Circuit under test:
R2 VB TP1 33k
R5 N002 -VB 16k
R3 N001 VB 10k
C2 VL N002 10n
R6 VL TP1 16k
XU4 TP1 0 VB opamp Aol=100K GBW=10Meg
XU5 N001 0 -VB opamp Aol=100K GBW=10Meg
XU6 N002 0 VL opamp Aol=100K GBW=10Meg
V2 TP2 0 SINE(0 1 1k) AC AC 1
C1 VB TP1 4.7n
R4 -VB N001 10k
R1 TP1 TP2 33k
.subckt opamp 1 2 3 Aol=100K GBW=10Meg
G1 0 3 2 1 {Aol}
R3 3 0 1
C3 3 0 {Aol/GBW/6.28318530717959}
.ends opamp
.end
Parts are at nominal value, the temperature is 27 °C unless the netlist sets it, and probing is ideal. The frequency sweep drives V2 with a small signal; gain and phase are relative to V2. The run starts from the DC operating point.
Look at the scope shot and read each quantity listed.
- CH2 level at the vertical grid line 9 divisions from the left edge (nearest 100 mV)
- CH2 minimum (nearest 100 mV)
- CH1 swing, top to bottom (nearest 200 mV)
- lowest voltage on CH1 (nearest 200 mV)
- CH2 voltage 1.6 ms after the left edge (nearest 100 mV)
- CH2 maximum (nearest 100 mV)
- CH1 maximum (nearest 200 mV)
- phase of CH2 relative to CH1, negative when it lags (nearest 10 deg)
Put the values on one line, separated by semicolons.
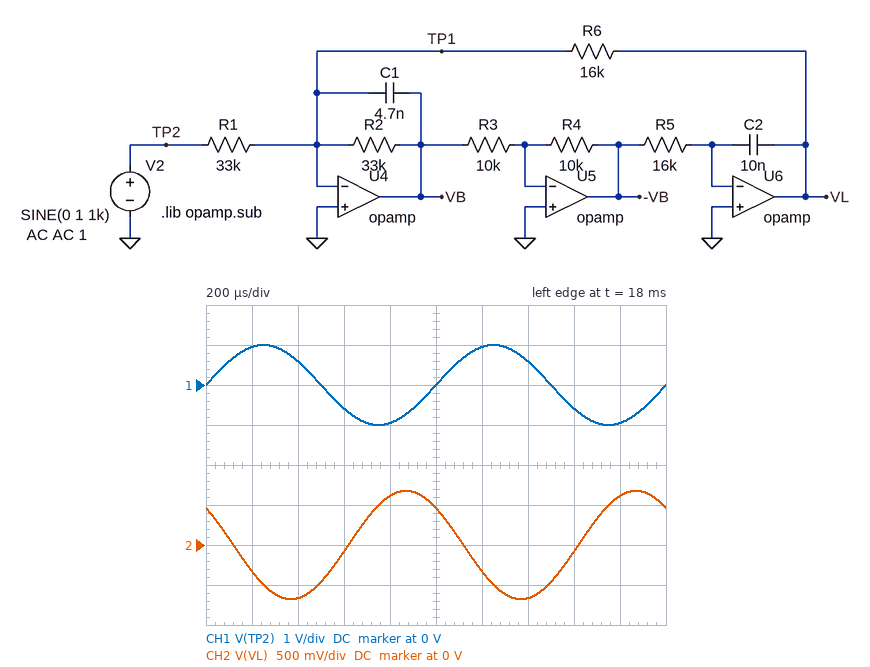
600 mV; -700 mV; 2.0 V; -1.0 V; -100 mV; 700 mV; 1.0 V; 140 deg
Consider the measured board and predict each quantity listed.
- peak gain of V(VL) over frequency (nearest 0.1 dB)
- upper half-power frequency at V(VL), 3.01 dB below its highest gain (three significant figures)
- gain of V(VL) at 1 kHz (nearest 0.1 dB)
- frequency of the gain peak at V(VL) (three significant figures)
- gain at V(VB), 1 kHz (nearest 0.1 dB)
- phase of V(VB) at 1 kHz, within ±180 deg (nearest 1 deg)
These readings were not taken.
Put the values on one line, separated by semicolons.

-2.7 dB; 1.72 kHz; -3.4 dB; 1.26 kHz; -3.3 dB; -133 deg
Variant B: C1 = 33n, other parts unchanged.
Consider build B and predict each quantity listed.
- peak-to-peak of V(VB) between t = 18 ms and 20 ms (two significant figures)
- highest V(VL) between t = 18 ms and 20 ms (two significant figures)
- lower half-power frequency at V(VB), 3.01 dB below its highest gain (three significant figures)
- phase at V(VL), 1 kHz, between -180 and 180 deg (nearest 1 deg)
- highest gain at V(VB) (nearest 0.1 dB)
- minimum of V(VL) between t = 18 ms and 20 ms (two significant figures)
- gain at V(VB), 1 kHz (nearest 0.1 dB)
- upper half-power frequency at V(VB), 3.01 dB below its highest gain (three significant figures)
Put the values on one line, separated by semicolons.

410 mV; 200 mV; 479 Hz; 12 deg; 0 dB; -200 mV; -13.8 dB; 625 Hz
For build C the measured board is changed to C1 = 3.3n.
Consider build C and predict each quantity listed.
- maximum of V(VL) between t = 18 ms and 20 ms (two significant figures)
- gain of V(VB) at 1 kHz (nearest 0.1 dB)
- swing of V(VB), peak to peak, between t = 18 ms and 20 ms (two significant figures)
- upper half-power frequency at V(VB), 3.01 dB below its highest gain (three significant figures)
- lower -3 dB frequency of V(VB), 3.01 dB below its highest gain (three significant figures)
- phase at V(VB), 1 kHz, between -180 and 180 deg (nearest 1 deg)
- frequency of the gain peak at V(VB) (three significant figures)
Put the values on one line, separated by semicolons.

590 mV; -4.6 dB; 1.2 V; 2.61 kHz; 1.15 kHz; -126 deg; 1.73 kHz
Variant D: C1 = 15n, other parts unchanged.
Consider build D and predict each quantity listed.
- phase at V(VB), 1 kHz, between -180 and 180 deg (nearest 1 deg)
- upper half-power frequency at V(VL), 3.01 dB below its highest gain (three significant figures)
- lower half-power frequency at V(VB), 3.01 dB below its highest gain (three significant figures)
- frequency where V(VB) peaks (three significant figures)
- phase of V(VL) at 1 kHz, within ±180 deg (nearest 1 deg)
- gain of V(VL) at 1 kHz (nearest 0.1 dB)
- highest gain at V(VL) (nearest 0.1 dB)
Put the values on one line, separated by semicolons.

133 deg; 929 Hz; 667 Hz; 812 Hz; 43 deg; -3.3 dB; 1.9 dB
